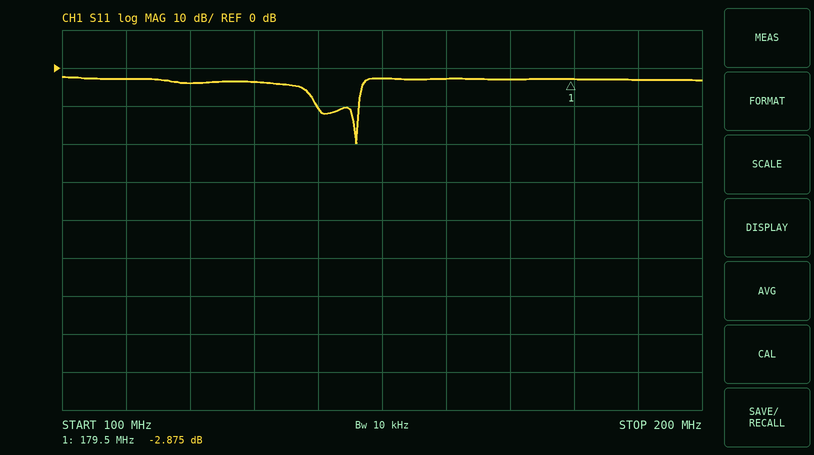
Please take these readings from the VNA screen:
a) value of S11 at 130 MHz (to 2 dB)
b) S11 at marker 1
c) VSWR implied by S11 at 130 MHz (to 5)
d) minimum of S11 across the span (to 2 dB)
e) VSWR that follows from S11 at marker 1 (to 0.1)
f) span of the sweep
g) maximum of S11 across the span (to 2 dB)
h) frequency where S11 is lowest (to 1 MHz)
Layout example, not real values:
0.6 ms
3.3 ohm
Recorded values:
-4 dB
-2.875 dB
5
-20 dB
6.1
100 MHz
-2 dB
146 MHz
